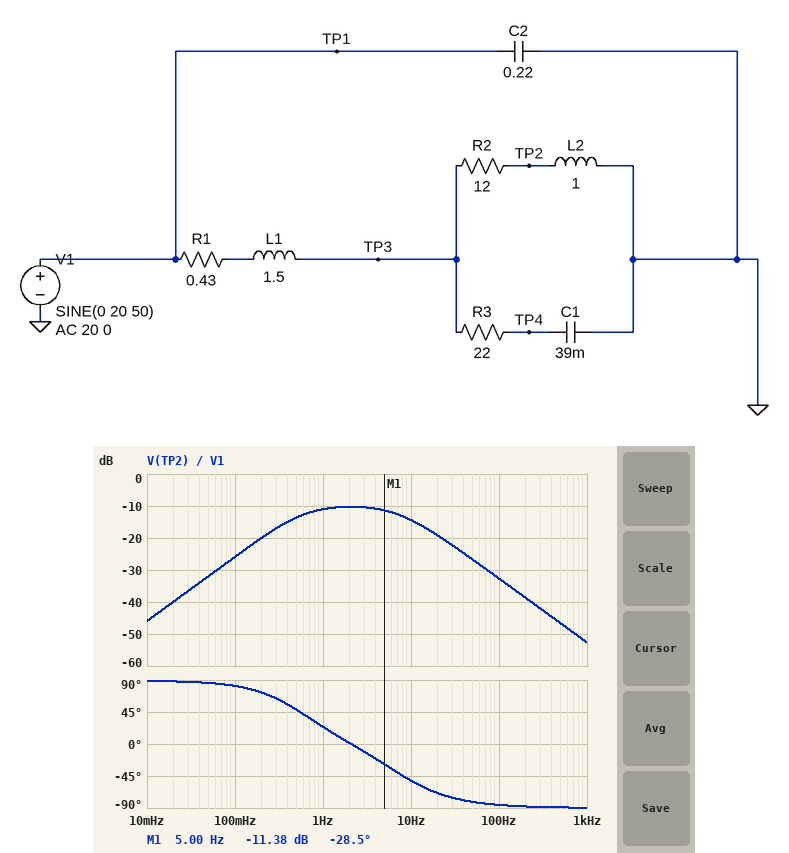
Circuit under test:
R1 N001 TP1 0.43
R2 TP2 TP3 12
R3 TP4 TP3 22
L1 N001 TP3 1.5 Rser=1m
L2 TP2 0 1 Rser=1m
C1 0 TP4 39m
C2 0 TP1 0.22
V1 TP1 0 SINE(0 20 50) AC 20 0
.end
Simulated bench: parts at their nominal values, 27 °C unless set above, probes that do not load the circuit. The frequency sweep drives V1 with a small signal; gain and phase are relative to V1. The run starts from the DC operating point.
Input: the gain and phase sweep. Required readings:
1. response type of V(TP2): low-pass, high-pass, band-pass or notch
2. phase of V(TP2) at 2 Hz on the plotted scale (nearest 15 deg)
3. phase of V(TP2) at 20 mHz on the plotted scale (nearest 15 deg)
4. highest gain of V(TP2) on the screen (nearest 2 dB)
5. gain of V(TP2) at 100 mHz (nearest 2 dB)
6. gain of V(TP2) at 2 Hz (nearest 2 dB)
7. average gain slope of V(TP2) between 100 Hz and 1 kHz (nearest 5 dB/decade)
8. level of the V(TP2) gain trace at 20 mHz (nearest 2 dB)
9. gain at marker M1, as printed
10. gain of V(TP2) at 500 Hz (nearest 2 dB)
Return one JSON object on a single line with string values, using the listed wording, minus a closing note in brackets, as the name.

{"response type of V(TP2): low-pass, high-pass, band-pass or notch": "band-pass", "phase of V(TP2) at 2 Hz on the plotted scale": "0 deg", "phase of V(TP2) at 20 mHz on the plotted scale": "90 deg", "highest gain of V(TP2) on the screen": "-10 dB", "gain of V(TP2) at 100 mHz": "-26 dB", "gain of V(TP2) at 2 Hz": "-10 dB", "average gain slope of V(TP2) between 100 Hz and 1 kHz": "-20 dB/decade", "level of the V(TP2) gain trace at 20 mHz": "-40 dB", "gain at marker M1, as printed": "-11.38 dB", "gain of V(TP2) at 500 Hz": "-46 dB"}
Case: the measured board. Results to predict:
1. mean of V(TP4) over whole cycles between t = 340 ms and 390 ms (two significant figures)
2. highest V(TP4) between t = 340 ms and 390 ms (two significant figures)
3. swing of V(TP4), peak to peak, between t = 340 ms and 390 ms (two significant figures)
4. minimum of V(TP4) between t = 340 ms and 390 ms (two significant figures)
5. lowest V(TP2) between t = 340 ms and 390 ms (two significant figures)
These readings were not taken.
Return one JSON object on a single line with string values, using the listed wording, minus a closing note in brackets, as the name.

{"mean of V(TP4) over whole cycles between t = 340 ms and 390 ms": "46 mV", "highest V(TP4) between t = 340 ms and 390 ms": "49 mV", "swing of V(TP4), peak to peak, between t = 340 ms and 390 ms": "7.0 mV", "minimum of V(TP4) between t = 340 ms and 390 ms": "42 mV", "lowest V(TP2) between t = 340 ms and 390 ms": "-950 mV"}
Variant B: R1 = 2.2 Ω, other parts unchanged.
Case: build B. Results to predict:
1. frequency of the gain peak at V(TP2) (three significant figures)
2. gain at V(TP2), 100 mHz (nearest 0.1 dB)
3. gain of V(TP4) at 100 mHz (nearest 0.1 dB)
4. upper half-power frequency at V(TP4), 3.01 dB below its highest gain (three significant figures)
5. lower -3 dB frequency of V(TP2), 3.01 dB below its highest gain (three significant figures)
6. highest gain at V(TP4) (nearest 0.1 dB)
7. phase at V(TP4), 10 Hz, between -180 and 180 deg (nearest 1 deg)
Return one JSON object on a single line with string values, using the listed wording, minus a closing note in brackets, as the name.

{"frequency of the gain peak at V(TP2)": "2.32 Hz", "gain at V(TP2), 100 mHz": "-27.2 dB", "gain of V(TP4) at 100 mHz": "-2.7 dB", "upper half-power frequency at V(TP4), 3.01 dB below its highest gain": "174 mHz", "lower -3 dB frequency of V(TP2), 3.01 dB below its highest gain": "637 mHz", "highest gain at V(TP4)": "-1.5 dB", "phase at V(TP4), 10 Hz, between -180 and 180 deg": "-150 deg"}
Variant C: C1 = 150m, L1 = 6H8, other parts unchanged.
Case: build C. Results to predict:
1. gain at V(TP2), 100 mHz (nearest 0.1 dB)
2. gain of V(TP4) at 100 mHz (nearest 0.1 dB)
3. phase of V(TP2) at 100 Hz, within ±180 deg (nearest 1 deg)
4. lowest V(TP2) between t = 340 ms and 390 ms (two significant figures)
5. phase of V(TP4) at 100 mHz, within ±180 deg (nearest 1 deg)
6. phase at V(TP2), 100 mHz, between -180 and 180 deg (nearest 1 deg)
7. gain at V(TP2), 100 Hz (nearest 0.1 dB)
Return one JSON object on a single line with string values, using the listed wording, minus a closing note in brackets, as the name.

{"gain at V(TP2), 100 mHz": "-26.6 dB", "gain of V(TP4) at 100 mHz": "-8.2 dB", "phase of V(TP2) at 100 Hz, within ±180 deg": "-87 deg", "lowest V(TP2) between t = 340 ms and 390 ms": "-210 mV", "phase of V(TP4) at 100 mHz, within ±180 deg": "-92 deg", "phase at V(TP2), 100 mHz, between -180 and 180 deg": "59 deg", "gain at V(TP2), 100 Hz": "-45.8 dB"}
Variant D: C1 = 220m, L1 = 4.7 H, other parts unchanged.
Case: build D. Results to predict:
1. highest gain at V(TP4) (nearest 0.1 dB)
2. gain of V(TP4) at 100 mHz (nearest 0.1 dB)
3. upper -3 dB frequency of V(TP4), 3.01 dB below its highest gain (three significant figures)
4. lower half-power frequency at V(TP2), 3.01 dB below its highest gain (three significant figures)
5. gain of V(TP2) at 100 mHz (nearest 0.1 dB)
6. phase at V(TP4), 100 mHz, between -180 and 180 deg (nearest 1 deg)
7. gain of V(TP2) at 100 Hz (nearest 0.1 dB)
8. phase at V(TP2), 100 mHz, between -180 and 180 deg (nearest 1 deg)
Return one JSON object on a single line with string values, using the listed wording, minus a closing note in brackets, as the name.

{"highest gain at V(TP4)": "-0.3 dB", "gain of V(TP4) at 100 mHz": "-10.9 dB", "upper -3 dB frequency of V(TP4), 3.01 dB below its highest gain": "33.2 mHz", "lower half-power frequency at V(TP2), 3.01 dB below its highest gain": "226 mHz", "gain of V(TP2) at 100 mHz": "-26.4 dB", "phase at V(TP4), 100 mHz, between -180 and 180 deg": "-92 deg", "gain of V(TP2) at 100 Hz": "-42.6 dB", "phase at V(TP2), 100 mHz, between -180 and 180 deg": "67 deg"}
